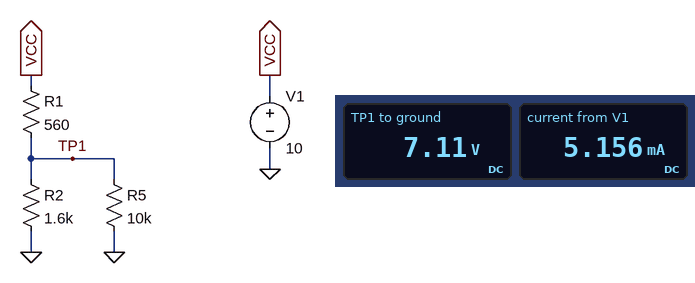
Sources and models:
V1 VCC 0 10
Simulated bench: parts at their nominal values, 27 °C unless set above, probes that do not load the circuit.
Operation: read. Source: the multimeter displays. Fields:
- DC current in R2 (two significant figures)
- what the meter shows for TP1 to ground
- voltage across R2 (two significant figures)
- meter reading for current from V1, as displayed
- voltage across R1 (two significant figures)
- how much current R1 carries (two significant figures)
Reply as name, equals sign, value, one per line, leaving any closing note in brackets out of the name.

DC current in R2 = 4.4 mA
what the meter shows for TP1 to ground = 7.11 V
voltage across R2 = 7.1 V
meter reading for current from V1, as displayed = 5.156 mA
voltage across R1 = 2.9 V
how much current R1 carries = 5.2 mA
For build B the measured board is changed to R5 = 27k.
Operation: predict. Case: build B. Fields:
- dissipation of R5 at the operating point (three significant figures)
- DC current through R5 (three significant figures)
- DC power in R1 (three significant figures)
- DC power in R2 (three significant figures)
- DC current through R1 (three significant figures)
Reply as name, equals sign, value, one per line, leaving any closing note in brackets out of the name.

dissipation of R5 at the operating point = 1.97 mW
DC current through R5 = 270 µA
DC power in R1 = 13.1 mW
DC power in R2 = 33.3 mW
DC current through R1 = 4.83 mA
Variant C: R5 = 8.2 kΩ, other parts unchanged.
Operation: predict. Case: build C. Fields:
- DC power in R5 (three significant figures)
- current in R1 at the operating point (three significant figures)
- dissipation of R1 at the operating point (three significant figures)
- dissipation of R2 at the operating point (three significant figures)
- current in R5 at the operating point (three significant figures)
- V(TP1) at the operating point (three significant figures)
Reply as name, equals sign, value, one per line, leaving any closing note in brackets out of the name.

DC power in R5 = 6.06 mW
current in R1 at the operating point = 5.27 mA
dissipation of R1 at the operating point = 15.5 mW
dissipation of R2 at the operating point = 31.1 mW
current in R5 at the operating point = 860 µA
V(TP1) at the operating point = 7.05 V
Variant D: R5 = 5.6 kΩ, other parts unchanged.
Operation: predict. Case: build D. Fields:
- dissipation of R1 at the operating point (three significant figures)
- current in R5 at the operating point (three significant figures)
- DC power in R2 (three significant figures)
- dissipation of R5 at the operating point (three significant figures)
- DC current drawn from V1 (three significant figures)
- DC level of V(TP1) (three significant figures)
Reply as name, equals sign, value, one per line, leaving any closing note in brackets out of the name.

dissipation of R1 at the operating point = 17.2 mW
current in R5 at the operating point = 1.23 mA
DC power in R2 = 29.7 mW
dissipation of R5 at the operating point = 8.49 mW
DC current drawn from V1 = 5.54 mA
DC level of V(TP1) = 6.90 V
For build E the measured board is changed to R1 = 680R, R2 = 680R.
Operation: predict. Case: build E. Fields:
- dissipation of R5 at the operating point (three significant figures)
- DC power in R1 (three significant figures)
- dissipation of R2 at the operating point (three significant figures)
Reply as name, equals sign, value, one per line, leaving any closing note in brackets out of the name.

dissipation of R5 at the operating point = 2.34 mW
DC power in R1 = 39.2 mW
dissipation of R2 at the operating point = 34.4 mW
